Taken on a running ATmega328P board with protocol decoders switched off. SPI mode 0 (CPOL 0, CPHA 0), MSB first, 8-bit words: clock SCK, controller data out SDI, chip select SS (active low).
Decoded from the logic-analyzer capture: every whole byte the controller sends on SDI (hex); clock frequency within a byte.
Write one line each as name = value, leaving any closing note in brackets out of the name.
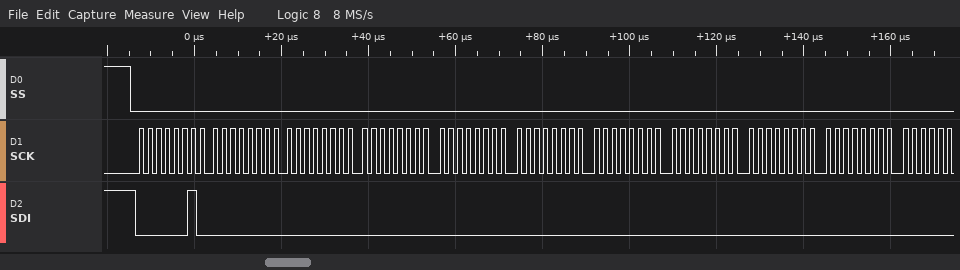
every whole byte the controller sends on SDI = 02 00 00 00 00 00 00 00 00 00
clock frequency within a byte = 500 kHz
